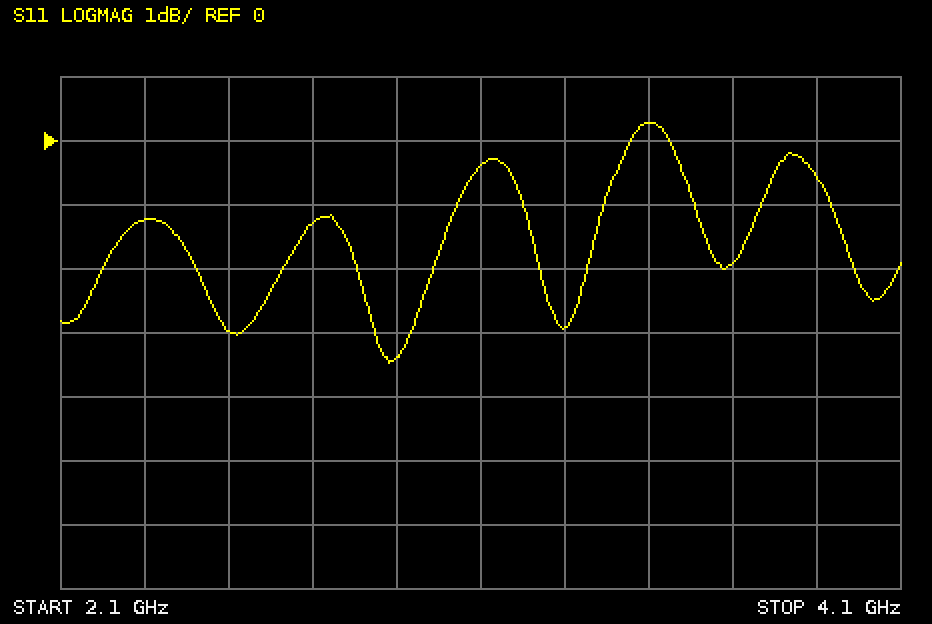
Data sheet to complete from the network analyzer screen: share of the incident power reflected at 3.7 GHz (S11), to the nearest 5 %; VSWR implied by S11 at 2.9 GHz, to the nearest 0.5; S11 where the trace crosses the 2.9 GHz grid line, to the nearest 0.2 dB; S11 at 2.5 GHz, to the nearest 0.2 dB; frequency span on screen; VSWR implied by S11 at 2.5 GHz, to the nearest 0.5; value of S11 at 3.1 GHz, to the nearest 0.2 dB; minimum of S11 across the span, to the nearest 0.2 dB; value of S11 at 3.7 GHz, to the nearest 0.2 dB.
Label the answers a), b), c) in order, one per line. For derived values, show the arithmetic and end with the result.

a) 10^(-2/10) ≈ 63.1 %, so 65 % to the nearest 5 %
b) |Γ| = 10^(-3.4/20) = 0.6761; VSWR = (1 + 0.6761)/(1 − 0.6761) ≈ 5.17, so 5.0 to the nearest 0.5
c) -3.4 dB
d) -3.0 dB
e) 2 GHz
f) |Γ| = 10^(-3/20) = 0.7079; VSWR = (1 + 0.7079)/(1 − 0.7079) ≈ 5.85, so 6.0 to the nearest 0.5
g) -0.4 dB
h) -3.4 dB
i) -2.0 dB
